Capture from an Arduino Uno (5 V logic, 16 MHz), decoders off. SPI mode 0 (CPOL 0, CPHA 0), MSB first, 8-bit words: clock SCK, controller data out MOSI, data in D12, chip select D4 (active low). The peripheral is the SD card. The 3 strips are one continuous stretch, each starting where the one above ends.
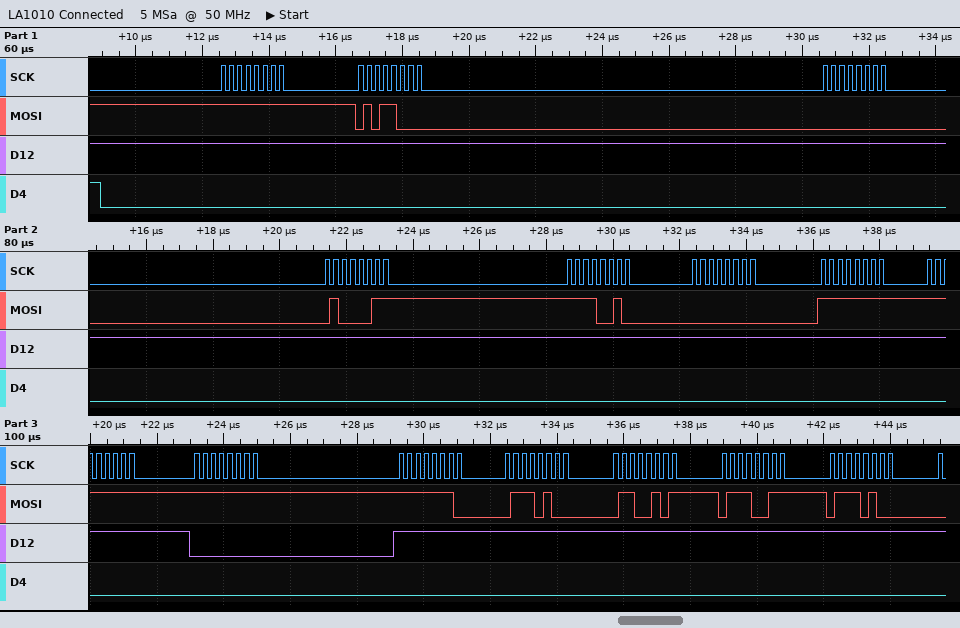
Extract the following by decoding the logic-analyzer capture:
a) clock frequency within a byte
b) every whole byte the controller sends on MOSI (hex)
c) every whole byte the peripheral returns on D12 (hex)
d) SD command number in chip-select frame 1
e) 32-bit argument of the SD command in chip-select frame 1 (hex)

4 MHz
FF 58 00 43 F2 00 FF FF FF FE 74 65 73 74
FF FF FF FF FF FF FF FF 00 FF FF FF FF FF
CMD24
0x0043F200
